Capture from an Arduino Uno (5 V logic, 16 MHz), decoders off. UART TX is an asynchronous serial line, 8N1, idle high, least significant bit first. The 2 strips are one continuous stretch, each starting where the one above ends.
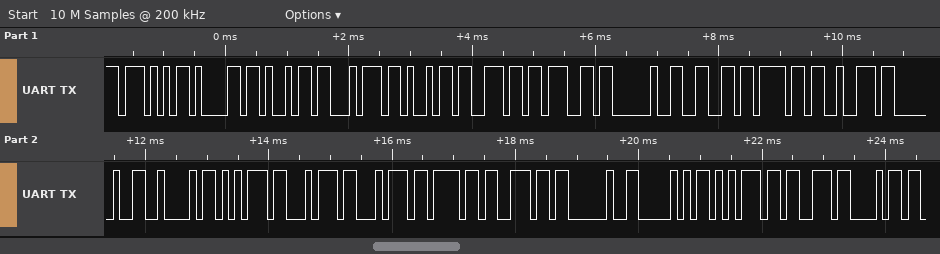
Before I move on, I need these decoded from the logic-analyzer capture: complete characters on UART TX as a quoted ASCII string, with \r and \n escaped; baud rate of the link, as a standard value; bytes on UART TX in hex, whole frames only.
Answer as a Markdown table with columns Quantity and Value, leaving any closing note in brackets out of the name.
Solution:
| Quantity | Value |
|---|---|
| complete characters on UART TX as a quoted ASCII string, with \r and \n escaped | "Waiting for Button Push" |
| baud rate of the link, as a standard value | 9600 baud |
| bytes on UART TX in hex, whole frames only | 57 61 69 74 69 6E 67 20 66 6F 72 20 42 75 74 74 6F 6E 20 50 75 73 68 |
